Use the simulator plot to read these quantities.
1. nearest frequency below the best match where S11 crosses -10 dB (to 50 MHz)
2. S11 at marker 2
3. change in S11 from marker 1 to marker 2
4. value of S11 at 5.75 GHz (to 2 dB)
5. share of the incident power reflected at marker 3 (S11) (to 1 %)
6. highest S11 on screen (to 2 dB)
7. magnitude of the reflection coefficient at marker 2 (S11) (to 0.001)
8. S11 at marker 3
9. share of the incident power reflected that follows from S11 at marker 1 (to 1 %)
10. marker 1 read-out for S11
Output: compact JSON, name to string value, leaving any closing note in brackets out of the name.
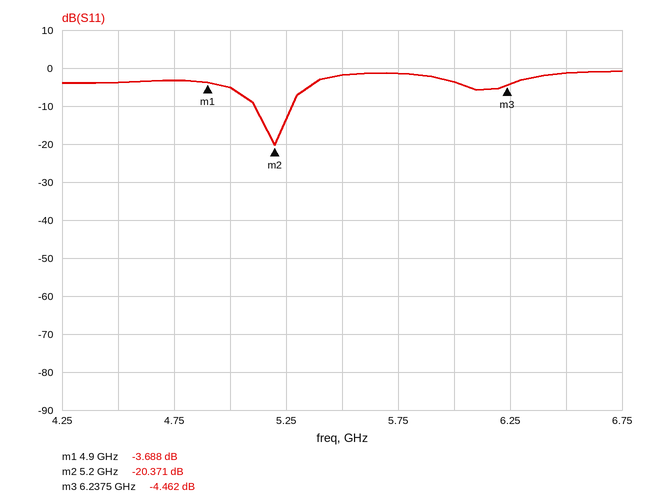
{"nearest frequency below the best match where S11 crosses -10 dB": "5.10 GHz", "S11 at marker 2": "-20.371 dB", "change in S11 from marker 1 to marker 2": "-16.683 dB", "value of S11 at 5.75 GHz": "-2 dB", "share of the incident power reflected at marker 3 (S11)": "36 %", "highest S11 on screen": "0 dB", "magnitude of the reflection coefficient at marker 2 (S11)": "0.096", "S11 at marker 3": "-4.462 dB", "share of the incident power reflected that follows from S11 at marker 1": "43 %", "marker 1 read-out for S11": "-3.688 dB"}
